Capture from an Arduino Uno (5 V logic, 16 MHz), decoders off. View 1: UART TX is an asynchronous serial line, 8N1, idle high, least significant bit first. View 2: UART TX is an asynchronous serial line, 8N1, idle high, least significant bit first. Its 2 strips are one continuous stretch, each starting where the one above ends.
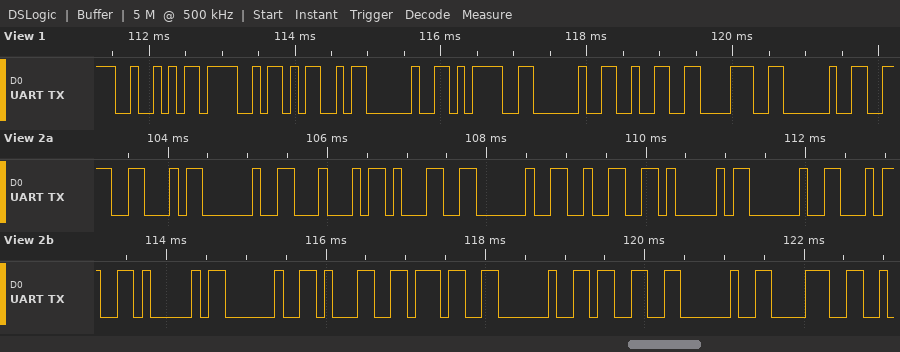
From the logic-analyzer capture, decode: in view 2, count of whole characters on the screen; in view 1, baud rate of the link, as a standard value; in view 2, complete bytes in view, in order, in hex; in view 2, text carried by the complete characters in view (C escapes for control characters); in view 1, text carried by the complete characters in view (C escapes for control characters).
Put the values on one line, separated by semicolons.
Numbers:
17; 9600 baud; 46 20 44 31 20 32 41 20 34 41 20 31 37 20 33 20 38; "F D1 2A 4A 17 3 8"; "ROM = 28 "
